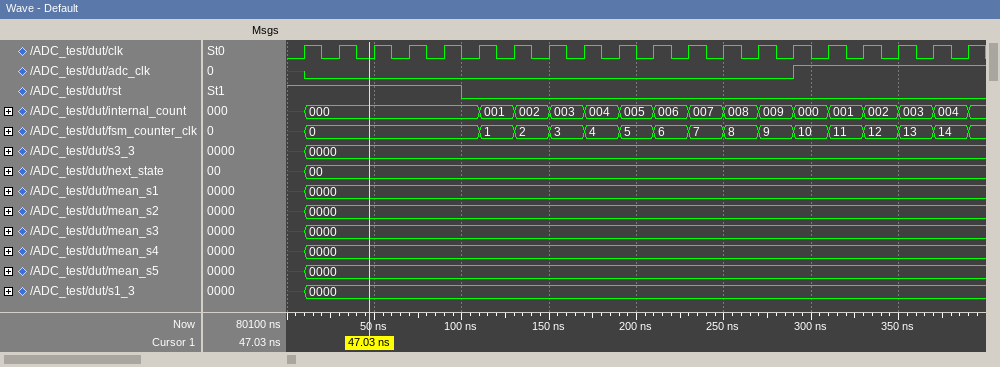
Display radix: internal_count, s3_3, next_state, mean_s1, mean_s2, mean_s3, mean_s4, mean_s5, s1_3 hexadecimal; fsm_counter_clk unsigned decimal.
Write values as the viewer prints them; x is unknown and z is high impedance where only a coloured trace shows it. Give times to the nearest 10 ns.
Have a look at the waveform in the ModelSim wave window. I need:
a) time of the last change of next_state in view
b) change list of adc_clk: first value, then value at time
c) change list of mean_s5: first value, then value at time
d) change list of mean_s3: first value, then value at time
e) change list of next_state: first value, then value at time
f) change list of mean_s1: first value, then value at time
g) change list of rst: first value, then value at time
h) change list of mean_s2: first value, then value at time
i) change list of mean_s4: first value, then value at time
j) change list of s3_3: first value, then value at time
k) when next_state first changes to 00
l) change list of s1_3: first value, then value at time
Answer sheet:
10 ns
x, 0 at 10 ns, 1 at 290 ns
x, 0000 at 10 ns
x, 0000 at 10 ns
x, 00 at 10 ns
x, 0000 at 10 ns
1, 0 at 100 ns
x, 0000 at 10 ns
x, 0000 at 10 ns
x, 0000 at 10 ns
10 ns
x, 0000 at 10 ns
